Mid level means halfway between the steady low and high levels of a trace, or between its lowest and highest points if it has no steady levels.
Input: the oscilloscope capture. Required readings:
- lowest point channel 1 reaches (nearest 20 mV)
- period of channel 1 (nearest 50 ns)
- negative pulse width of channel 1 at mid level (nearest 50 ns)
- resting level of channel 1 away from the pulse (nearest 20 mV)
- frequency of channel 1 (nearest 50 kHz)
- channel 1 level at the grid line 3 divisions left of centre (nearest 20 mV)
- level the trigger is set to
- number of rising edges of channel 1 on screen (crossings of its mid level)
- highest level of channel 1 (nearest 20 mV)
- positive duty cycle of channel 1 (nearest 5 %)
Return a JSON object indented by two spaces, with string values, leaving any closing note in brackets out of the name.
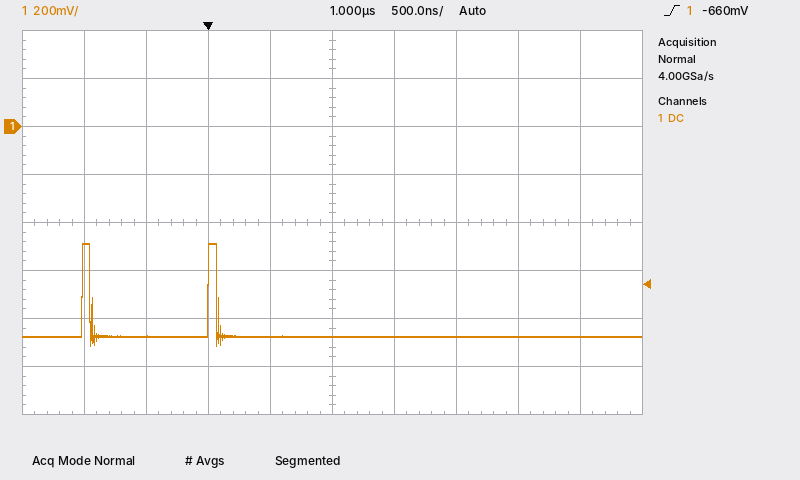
{
  "lowest point channel 1 reaches": "-920 mV",
  "period of channel 1": "1.00 µs",
  "negative pulse width of channel 1 at mid level": "950 ns",
  "resting level of channel 1 away from the pulse": "-880 mV",
  "frequency of channel 1": "1.00 MHz",
  "channel 1 level at the grid line 3 divisions left of centre": "-880 mV",
  "level the trigger is set to": "-660 mV",
  "number of rising edges of channel 1 on screen": "2",
  "highest level of channel 1": "-480 mV",
  "positive duty cycle of channel 1": "5 %"
}
